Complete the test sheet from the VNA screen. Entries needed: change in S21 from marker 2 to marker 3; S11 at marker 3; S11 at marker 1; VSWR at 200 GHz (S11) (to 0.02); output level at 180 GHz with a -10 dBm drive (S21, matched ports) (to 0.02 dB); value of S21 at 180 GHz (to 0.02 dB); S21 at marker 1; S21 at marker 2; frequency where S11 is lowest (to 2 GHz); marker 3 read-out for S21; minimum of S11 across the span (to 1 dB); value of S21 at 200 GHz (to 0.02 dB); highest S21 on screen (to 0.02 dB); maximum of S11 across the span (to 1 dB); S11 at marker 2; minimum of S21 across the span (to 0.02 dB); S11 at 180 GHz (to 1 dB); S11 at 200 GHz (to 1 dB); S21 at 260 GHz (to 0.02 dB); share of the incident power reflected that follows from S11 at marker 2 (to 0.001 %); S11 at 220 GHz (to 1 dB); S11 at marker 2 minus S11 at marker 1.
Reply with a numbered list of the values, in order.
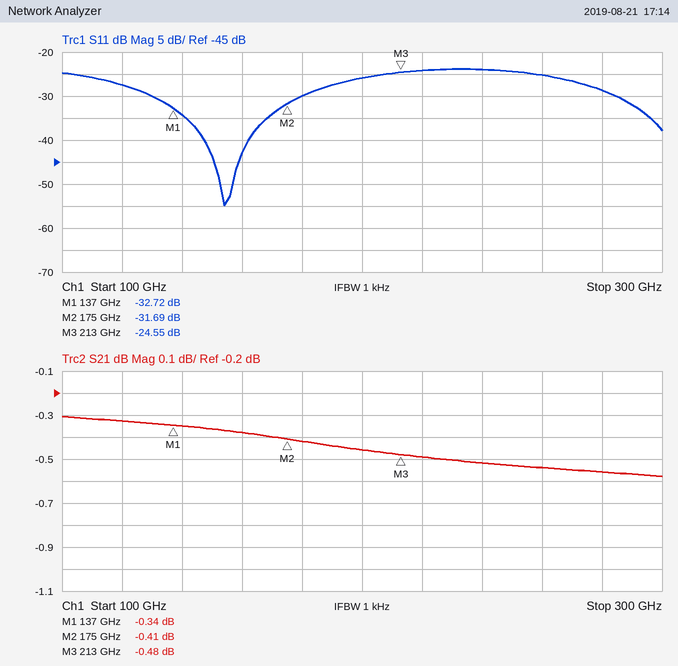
1. -0.07 dB
2. -24.55 dB
3. -32.72 dB
4. 1.10
5. -10.42 dBm
6. -0.42 dB
7. -0.34 dB
8. -0.41 dB
9. 154 GHz
10. -0.48 dB
11. -55 dB
12. -0.46 dB
13. -0.30 dB
14. -24 dB
15. -31.69 dB
16. -0.58 dB
17. -30 dB
18. -26 dB
19. -0.54 dB
20. 0.068 %
21. -24 dB
22. 1.03 dB
